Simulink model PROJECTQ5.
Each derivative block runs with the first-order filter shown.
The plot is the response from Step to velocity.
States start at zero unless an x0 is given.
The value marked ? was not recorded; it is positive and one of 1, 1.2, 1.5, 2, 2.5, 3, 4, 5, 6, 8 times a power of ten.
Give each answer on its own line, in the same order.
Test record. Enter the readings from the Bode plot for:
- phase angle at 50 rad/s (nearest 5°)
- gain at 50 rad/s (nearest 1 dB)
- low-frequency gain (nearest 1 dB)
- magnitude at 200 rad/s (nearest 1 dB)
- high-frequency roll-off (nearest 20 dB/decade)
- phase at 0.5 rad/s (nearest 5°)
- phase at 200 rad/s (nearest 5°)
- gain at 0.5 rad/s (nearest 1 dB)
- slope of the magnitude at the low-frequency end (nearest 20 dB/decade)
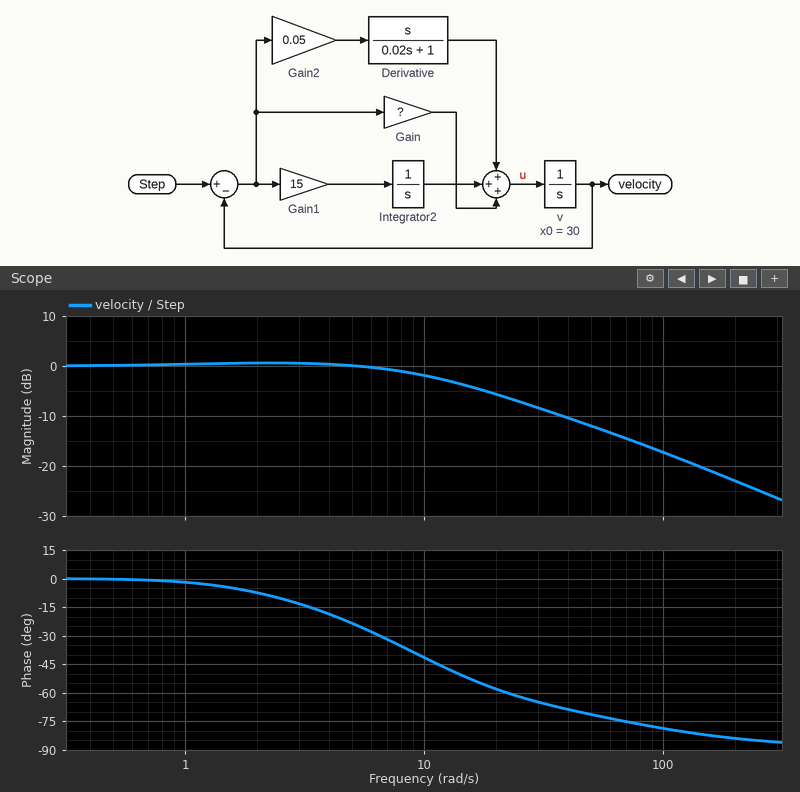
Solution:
-70°
-12 dB
0 dB
-23 dB
-20 dB/decade
0°
-85°
0 dB
0 dB/decade
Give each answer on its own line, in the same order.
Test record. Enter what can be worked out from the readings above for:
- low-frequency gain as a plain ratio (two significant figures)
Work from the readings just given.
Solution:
1.0
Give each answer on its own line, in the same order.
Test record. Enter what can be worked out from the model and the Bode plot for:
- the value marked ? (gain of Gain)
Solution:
12
